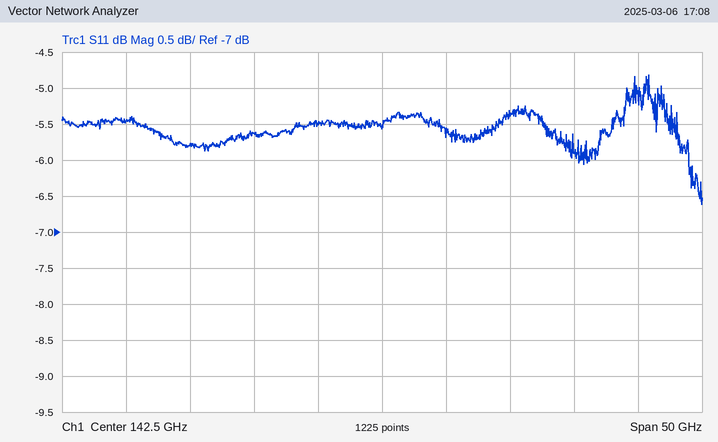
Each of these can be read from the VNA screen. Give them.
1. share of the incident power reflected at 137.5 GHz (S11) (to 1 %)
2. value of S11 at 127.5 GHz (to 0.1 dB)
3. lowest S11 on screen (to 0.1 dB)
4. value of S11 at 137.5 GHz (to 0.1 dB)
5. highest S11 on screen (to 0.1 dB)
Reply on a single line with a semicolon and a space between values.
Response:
28 %; -5.8 dB; -6.6 dB; -5.5 dB; -4.8 dB
